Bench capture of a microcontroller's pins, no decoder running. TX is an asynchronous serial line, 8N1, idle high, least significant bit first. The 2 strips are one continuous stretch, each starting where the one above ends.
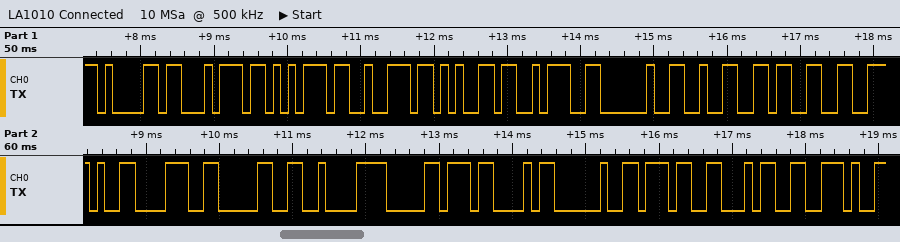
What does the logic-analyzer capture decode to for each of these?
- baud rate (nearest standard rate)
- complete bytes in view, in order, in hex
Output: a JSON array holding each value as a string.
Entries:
["9600 baud", "0x61 0x74 0x75 0x72 0x65 0x3A 0x20 0x32 0x33 0x2E 0x38 0x30 0xC2 0xB0 0x43 0x20 0x37 0x34 0x2E"]
